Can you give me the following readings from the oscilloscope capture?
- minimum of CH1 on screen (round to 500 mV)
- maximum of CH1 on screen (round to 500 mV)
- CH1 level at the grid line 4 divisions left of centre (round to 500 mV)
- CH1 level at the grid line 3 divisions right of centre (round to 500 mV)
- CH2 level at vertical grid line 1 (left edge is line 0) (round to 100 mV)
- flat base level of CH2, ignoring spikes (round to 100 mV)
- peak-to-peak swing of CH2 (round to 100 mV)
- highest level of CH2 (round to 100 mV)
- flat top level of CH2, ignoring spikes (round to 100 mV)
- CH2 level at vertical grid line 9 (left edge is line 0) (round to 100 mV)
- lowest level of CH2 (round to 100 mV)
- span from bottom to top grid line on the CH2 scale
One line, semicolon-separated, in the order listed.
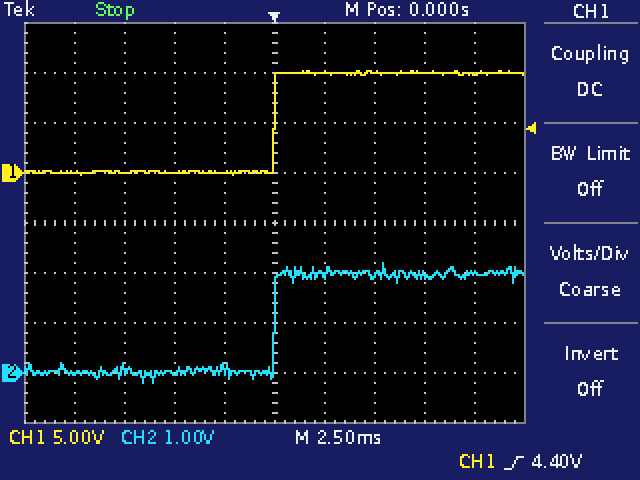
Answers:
0.0 V; 10.0 V; 0.0 V; 10.0 V; 0.0 V; 0.0 V; 2.4 V; 2.2 V; 2.0 V; 2.0 V; -200 mV; 8 V
